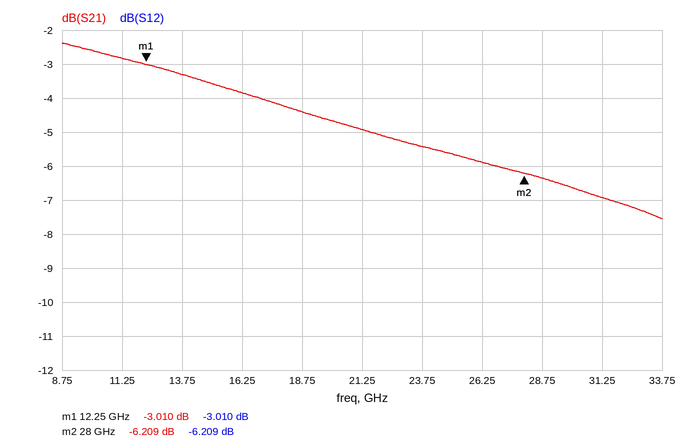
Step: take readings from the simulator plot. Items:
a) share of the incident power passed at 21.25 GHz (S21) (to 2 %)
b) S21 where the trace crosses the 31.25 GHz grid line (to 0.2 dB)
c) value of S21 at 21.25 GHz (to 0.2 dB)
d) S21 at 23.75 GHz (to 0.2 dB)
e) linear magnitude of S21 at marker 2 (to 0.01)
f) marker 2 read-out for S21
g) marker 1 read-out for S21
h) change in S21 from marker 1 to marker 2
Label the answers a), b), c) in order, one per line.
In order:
a) 32 %
b) -7.0 dB
c) -5.0 dB
d) -5.4 dB
e) 0.49
f) -6.209 dB
g) -3.010 dB
h) -3.199 dB
